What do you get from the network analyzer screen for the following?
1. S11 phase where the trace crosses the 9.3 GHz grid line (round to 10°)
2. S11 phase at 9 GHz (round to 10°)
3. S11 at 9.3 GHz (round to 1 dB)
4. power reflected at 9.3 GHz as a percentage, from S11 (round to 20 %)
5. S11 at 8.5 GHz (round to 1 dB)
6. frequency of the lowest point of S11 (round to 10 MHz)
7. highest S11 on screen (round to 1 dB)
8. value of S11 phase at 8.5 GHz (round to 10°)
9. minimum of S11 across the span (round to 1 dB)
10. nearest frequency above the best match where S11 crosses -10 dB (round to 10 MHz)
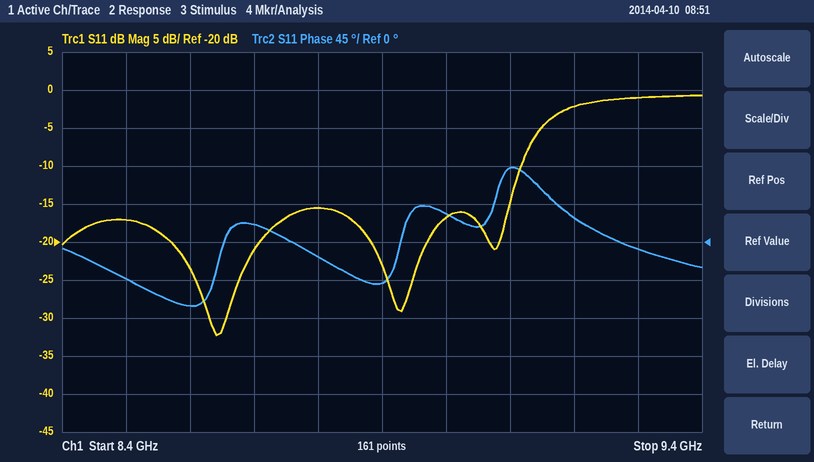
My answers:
-10°
30°
-1 dB
80 %
-17 dB
8.64 GHz
-1 dB
-40°
-32 dB
9.12 GHz
